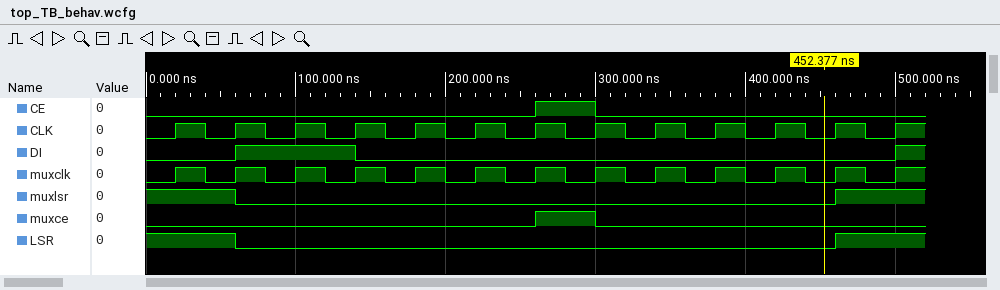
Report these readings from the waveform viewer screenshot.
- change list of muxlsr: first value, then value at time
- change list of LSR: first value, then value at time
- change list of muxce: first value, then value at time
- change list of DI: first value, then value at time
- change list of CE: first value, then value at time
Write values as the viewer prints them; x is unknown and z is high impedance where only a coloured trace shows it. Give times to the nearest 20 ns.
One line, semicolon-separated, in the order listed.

1, 0 at 60 ns, 1 at 460 ns; 1, 0 at 60 ns, 1 at 460 ns; 0, 1 at 260 ns, 0 at 300 ns; 0, 1 at 60 ns, 0 at 140 ns, 1 at 500 ns; 0, 1 at 260 ns, 0 at 300 ns
